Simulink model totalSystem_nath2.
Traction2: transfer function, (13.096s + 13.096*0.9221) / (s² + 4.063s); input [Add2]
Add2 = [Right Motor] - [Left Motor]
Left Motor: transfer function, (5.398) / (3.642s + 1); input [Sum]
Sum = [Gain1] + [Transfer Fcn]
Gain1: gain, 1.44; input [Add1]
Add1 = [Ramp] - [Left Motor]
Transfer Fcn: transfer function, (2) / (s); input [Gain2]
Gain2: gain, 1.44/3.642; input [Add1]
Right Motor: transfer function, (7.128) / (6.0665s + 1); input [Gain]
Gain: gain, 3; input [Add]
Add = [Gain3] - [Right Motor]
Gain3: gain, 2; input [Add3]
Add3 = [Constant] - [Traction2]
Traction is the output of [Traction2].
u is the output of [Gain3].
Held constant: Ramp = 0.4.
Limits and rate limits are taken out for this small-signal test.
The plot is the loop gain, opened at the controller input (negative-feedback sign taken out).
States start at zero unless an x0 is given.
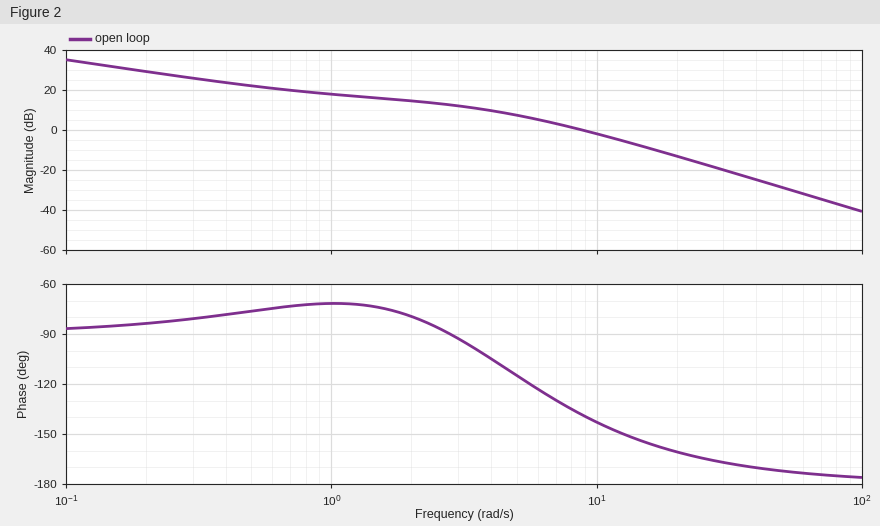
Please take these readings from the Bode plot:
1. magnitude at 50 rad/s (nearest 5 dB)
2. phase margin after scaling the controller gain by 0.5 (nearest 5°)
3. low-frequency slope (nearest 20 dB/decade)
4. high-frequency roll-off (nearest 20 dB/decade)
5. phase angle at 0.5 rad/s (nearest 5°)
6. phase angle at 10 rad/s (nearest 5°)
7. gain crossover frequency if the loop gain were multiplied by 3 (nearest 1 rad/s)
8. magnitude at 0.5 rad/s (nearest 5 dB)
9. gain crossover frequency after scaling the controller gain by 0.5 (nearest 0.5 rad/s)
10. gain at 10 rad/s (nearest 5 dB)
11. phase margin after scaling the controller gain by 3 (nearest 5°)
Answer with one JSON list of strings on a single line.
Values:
["-30 dB", "60°", "-20 dB/decade", "-40 dB/decade", "-75°", "-145°", "16 rad/s", "20 dB", "5.5 rad/s", "0 dB", "25°"]
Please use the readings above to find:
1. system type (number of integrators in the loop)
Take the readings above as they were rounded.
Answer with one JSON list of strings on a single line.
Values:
["1"]
